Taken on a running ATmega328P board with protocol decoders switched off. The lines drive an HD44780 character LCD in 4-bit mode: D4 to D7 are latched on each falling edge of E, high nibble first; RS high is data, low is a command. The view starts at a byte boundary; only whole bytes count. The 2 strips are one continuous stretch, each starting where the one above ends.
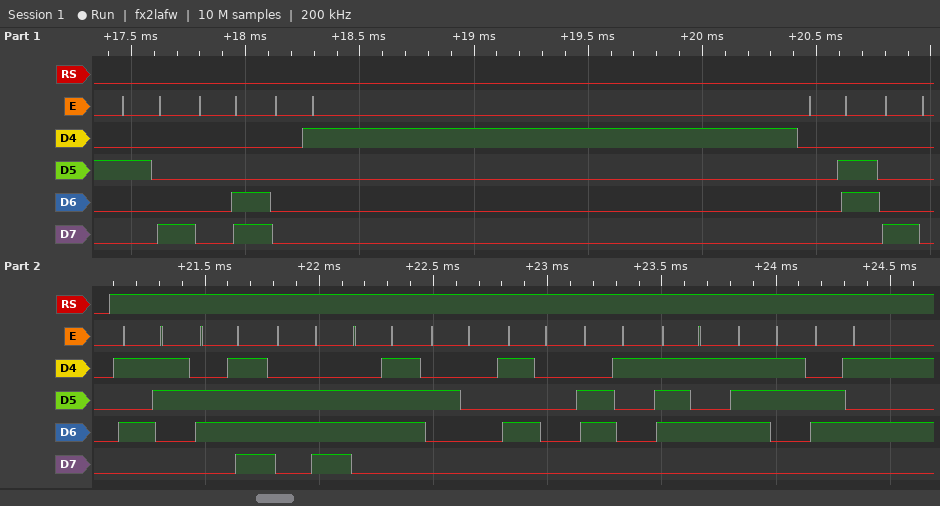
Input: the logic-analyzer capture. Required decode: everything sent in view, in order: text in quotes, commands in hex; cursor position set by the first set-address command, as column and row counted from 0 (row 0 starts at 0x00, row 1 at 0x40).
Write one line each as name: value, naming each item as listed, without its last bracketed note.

everything sent in view, in order: text in quotes, commands in hex: 0x28 0x0C 0x01 0x06 0x80 "Song Pause"
cursor position set by the first set-address command, as column and row counted from 0: column 0, row 0
